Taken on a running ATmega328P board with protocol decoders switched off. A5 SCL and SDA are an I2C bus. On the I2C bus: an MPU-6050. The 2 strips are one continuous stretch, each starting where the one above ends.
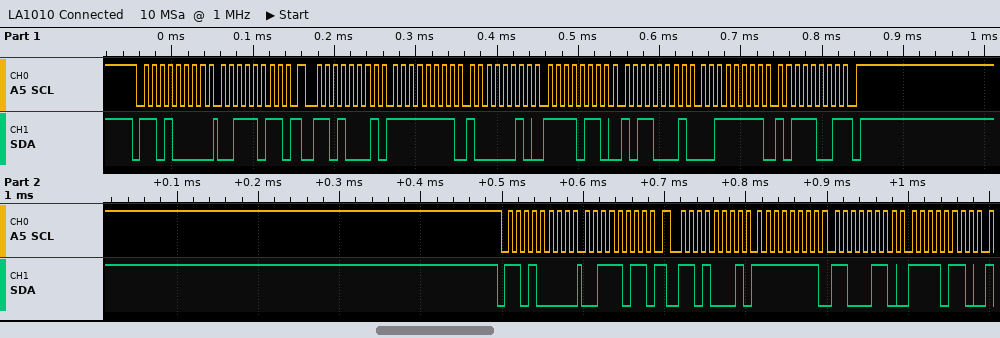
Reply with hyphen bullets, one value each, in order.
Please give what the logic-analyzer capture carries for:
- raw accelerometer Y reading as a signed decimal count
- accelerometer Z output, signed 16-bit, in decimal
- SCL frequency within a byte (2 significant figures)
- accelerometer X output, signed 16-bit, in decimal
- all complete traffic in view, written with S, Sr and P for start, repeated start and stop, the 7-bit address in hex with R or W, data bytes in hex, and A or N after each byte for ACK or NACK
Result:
- -2383
- 16313
- 100 kHz
- -126
- S 68W A 3B A Sr 68R A FF A 82 A F6 A B1 A 3F A B9 N P S 68W A 3B A Sr 68R A FF A C6 A F6 A
